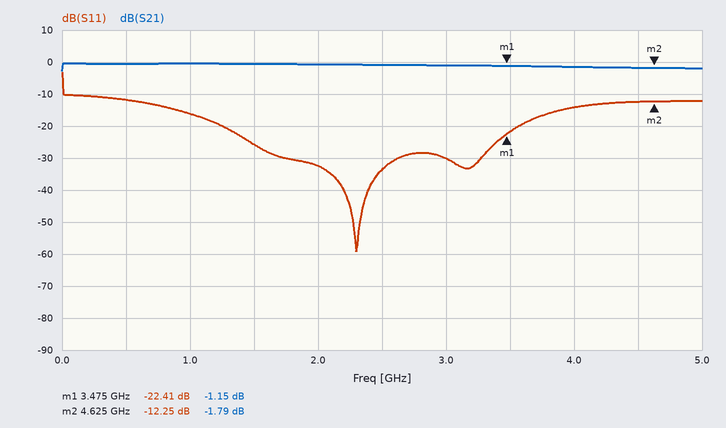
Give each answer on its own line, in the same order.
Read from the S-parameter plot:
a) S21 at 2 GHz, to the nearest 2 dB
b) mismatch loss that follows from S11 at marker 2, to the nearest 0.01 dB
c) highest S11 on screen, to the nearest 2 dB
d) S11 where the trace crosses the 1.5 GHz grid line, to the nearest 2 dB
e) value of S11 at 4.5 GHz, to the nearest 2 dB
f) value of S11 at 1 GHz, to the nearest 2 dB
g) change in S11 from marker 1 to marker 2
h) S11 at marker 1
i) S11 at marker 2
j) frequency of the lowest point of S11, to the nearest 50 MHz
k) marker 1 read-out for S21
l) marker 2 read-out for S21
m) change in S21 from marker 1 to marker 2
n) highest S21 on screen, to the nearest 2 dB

0 dB
0.27 dB
-4 dB
-26 dB
-12 dB
-16 dB
10.16 dB
-22.41 dB
-12.25 dB
2.30 GHz
-1.15 dB
-1.79 dB
-0.64 dB
0 dB
